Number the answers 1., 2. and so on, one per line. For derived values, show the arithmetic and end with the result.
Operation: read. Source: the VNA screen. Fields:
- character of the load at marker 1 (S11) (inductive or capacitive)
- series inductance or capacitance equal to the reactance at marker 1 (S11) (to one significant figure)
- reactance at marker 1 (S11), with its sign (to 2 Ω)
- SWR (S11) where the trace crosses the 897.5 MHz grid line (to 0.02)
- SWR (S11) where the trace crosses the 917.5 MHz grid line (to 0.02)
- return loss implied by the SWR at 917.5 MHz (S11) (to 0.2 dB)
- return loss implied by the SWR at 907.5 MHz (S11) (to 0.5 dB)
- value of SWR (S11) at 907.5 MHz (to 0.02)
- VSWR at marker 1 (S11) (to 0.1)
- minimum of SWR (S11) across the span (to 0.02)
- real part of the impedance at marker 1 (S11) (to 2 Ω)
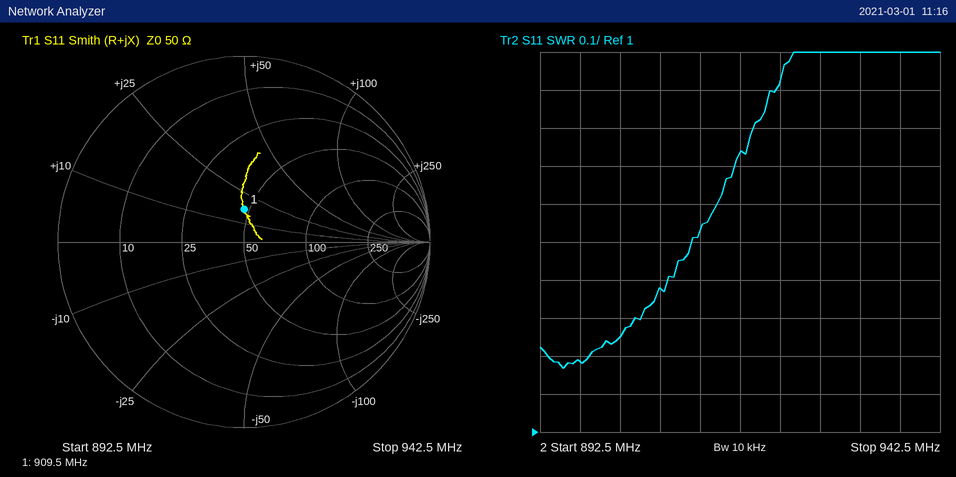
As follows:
1. inductive
2. L = 18 Ω/(2π × 909.5 MHz) ≈ 3 nH
3. +18 Ω
4. 1.18
5. 1.74
6. −20 log10((1.74 − 1)/(1.74 + 1)) ≈ 11.4 dB
7. −20 log10((1.38 − 1)/(1.38 + 1)) ≈ 15.9 dB, so 16.0 dB to the nearest 0.5 dB
8. 1.38
9. 1.4
10. 1.16
11. 48 Ω
